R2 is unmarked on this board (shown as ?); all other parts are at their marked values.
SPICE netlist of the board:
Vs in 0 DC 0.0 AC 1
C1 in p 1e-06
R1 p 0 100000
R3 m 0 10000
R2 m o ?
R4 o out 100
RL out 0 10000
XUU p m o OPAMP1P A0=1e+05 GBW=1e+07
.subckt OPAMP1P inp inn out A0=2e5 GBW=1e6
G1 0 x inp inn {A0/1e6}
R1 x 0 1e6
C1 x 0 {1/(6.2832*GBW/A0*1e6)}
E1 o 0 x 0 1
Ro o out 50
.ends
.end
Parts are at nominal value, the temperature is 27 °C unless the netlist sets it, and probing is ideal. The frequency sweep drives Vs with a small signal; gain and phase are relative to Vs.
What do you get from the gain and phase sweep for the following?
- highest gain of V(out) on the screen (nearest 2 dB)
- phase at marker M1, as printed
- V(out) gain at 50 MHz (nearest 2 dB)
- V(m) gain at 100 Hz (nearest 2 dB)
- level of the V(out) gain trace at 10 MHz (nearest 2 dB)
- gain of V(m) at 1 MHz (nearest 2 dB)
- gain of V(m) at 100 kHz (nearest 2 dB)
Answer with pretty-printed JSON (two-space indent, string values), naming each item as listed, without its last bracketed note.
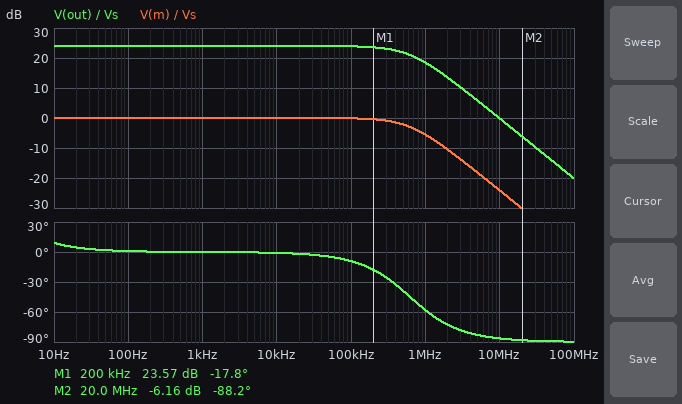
{
  "highest gain of V(out) on the screen": "24 dB",
  "phase at marker M1, as printed": "-17.8 deg",
  "V(out) gain at 50 MHz": "-14 dB",
  "V(m) gain at 100 Hz": "0 dB",
  "level of the V(out) gain trace at 10 MHz": "0 dB",
  "gain of V(m) at 1 MHz": "-6 dB",
  "gain of V(m) at 100 kHz": "0 dB"
}
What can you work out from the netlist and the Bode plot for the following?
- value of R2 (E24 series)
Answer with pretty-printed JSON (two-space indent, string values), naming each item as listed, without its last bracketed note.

{
  "value of R2": "150 kΩ"
}
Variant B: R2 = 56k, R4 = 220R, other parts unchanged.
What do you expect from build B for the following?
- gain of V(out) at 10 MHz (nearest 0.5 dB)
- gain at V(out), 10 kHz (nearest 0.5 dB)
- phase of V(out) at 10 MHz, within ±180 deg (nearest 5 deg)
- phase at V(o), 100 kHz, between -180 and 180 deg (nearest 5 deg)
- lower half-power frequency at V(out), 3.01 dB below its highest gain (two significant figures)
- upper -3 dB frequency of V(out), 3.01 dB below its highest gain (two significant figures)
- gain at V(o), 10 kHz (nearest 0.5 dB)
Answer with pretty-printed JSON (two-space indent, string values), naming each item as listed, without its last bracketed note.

{
  "gain of V(out) at 10 MHz": "-0.5 dB",
  "gain at V(out), 10 kHz": "16.0 dB",
  "phase of V(out) at 10 MHz, within ±180 deg": "-80 deg",
  "phase at V(o), 100 kHz, between -180 and 180 deg": "-5 deg",
  "lower half-power frequency at V(out), 3.01 dB below its highest gain": "1.6 Hz",
  "upper -3 dB frequency of V(out), 3.01 dB below its highest gain": "1.5 MHz",
  "gain at V(o), 10 kHz": "16.5 dB"
}
